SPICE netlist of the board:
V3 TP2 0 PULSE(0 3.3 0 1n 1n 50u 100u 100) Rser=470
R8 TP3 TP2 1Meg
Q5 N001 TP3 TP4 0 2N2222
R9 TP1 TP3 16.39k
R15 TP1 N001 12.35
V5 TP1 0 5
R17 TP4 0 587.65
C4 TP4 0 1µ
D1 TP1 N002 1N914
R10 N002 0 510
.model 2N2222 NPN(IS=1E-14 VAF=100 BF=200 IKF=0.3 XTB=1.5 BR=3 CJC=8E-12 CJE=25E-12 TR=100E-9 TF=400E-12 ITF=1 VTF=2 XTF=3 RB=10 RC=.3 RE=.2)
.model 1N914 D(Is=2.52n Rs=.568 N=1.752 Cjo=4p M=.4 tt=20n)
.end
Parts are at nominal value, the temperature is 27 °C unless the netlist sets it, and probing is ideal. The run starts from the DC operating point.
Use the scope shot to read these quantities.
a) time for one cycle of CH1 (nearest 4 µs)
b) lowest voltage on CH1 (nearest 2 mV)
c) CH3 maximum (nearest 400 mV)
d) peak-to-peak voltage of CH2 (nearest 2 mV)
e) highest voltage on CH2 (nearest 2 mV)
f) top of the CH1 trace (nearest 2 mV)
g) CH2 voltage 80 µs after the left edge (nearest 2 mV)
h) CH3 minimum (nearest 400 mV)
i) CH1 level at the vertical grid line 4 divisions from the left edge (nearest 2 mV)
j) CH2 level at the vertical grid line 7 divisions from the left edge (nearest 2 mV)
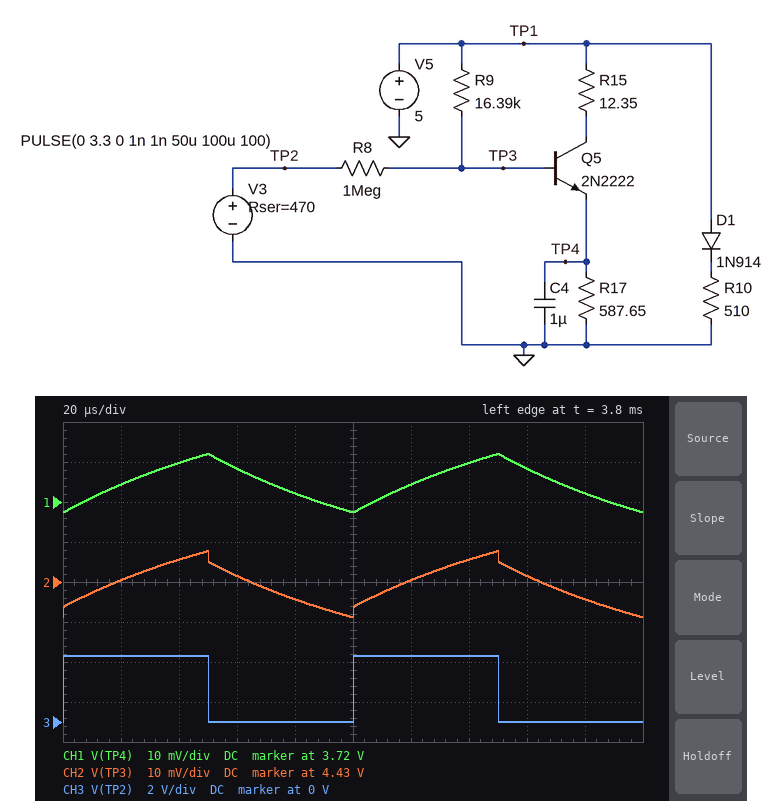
100 µs
3.718 V
3.2 V
16 mV
4.438 V
3.732 V
4.426 V
0 V
3.722 V
4.436 V
